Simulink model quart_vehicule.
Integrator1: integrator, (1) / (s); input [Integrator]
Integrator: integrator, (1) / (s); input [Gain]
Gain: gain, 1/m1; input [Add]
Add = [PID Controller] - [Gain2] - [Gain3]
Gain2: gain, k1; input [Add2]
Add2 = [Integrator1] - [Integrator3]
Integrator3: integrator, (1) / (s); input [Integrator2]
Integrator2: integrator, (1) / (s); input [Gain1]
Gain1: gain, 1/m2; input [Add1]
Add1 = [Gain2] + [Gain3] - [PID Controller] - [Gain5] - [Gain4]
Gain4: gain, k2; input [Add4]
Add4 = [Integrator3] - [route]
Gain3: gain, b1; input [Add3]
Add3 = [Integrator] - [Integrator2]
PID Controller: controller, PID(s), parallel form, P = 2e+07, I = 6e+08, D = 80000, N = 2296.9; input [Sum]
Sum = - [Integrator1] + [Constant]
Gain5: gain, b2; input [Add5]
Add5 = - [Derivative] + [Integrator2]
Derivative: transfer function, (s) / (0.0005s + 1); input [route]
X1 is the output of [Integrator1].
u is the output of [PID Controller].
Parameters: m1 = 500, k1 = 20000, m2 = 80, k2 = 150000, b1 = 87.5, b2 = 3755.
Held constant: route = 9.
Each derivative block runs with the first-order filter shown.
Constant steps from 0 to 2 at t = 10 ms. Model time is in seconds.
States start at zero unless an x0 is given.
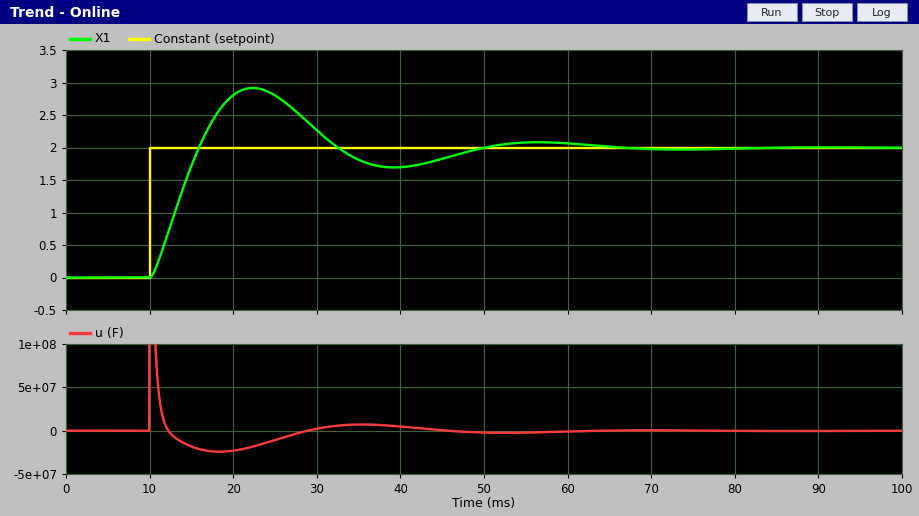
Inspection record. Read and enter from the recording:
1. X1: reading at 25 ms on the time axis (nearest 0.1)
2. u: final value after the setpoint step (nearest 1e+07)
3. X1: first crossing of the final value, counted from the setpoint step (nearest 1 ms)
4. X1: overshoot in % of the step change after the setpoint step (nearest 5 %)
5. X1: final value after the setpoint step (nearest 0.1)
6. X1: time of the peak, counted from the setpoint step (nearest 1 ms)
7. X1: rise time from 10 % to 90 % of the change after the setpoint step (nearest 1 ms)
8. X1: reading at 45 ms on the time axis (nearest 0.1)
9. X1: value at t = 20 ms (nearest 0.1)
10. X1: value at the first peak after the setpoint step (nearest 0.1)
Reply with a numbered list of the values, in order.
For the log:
1. 2.8
2. 0
3. 6 ms
4. 45 %
5. 2.0
6. 12 ms
7. 4 ms
8. 1.8
9. 2.8
10. 2.9
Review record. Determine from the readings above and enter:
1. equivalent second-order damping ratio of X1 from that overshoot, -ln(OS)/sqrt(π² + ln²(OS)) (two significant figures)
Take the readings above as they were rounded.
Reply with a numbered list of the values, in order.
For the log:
1. 0.25
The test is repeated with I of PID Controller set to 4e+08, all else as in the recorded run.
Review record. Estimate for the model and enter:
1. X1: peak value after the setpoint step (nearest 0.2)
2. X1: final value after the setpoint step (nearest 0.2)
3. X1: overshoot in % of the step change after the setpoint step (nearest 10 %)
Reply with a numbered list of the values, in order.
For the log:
1. 2.8
2. 2.0
3. 40 %
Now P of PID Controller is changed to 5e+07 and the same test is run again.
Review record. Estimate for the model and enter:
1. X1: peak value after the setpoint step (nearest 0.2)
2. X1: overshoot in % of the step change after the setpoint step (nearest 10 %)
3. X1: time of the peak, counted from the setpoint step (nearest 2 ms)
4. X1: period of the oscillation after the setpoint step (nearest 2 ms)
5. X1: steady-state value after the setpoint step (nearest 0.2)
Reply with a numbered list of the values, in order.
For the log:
1. 3.2
2. 60 %
3. 8 ms
4. 20 ms
5. 2.0
